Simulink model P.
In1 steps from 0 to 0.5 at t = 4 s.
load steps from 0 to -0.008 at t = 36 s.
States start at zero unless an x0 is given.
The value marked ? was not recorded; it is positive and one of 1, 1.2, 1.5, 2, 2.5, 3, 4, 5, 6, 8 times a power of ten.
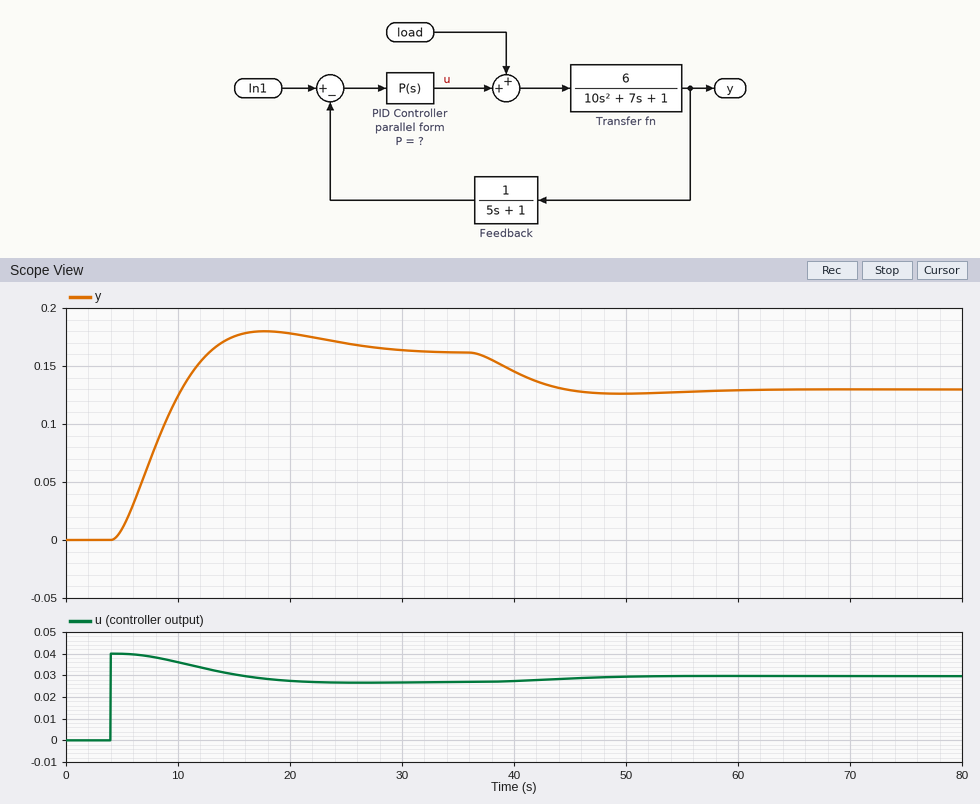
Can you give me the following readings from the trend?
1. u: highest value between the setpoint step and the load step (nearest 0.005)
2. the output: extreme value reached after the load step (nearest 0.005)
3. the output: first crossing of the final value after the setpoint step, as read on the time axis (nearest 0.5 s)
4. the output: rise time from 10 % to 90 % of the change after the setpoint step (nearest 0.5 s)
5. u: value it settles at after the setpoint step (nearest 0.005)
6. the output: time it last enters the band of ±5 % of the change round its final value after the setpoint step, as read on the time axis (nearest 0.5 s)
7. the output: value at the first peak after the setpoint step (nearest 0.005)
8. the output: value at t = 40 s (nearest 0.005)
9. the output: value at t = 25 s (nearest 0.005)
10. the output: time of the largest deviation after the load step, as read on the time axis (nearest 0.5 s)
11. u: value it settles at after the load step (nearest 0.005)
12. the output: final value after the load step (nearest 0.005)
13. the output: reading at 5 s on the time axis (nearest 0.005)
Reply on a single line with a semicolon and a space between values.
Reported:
0.040; 0.125; 13.0 s; 6.0 s; 0.025; 24.5 s; 0.180; 0.145; 0.170; 49.5 s; 0.030; 0.130; 0.010
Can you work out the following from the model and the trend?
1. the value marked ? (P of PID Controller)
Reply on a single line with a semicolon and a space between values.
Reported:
0.08
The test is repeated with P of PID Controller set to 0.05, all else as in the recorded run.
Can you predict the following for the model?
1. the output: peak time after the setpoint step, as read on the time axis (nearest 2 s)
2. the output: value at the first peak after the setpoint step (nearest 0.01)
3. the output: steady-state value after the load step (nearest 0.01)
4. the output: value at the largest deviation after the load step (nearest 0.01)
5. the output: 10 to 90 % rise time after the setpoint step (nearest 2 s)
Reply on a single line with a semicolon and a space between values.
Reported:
20 s; 0.12; 0.08; 0.08; 8 s
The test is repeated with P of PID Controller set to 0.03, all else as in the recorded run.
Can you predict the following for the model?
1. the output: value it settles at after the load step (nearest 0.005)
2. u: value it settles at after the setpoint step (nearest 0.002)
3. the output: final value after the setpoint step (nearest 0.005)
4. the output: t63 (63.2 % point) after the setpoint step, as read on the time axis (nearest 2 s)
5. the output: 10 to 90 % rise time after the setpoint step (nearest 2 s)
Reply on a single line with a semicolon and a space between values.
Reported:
0.035; 0.012; 0.075; 10 s; 8 s
